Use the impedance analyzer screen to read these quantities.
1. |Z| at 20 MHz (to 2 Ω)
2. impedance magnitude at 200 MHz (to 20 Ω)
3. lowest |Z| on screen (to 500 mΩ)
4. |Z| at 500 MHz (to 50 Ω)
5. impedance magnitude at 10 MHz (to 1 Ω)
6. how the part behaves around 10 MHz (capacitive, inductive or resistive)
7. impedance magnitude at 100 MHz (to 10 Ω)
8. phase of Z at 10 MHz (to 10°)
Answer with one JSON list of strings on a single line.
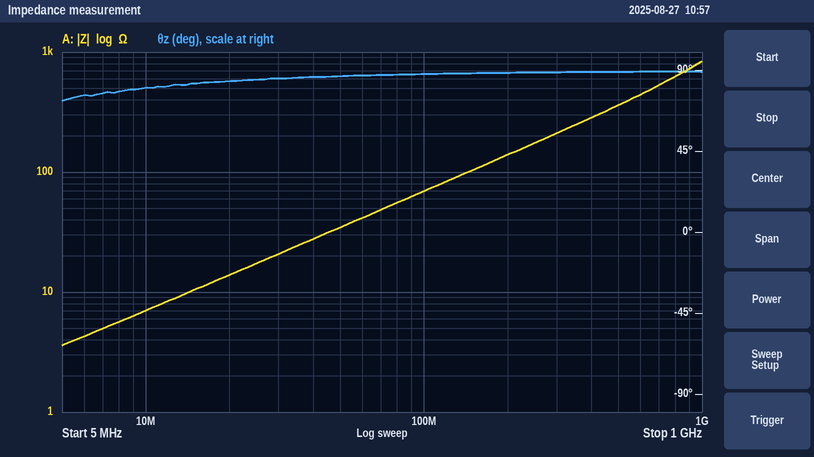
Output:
["14 Ω", "140 Ω", "3.5 Ω", "350 Ω", "7 Ω", "inductive", "70 Ω", "80°"]
